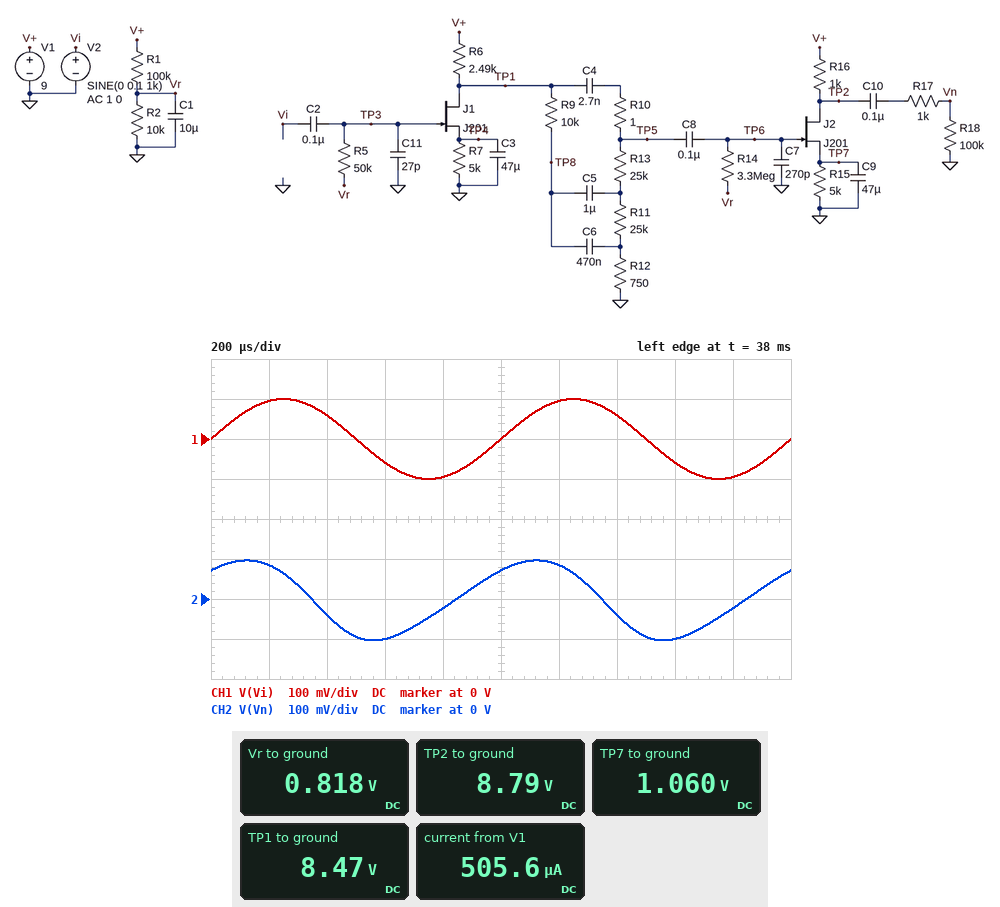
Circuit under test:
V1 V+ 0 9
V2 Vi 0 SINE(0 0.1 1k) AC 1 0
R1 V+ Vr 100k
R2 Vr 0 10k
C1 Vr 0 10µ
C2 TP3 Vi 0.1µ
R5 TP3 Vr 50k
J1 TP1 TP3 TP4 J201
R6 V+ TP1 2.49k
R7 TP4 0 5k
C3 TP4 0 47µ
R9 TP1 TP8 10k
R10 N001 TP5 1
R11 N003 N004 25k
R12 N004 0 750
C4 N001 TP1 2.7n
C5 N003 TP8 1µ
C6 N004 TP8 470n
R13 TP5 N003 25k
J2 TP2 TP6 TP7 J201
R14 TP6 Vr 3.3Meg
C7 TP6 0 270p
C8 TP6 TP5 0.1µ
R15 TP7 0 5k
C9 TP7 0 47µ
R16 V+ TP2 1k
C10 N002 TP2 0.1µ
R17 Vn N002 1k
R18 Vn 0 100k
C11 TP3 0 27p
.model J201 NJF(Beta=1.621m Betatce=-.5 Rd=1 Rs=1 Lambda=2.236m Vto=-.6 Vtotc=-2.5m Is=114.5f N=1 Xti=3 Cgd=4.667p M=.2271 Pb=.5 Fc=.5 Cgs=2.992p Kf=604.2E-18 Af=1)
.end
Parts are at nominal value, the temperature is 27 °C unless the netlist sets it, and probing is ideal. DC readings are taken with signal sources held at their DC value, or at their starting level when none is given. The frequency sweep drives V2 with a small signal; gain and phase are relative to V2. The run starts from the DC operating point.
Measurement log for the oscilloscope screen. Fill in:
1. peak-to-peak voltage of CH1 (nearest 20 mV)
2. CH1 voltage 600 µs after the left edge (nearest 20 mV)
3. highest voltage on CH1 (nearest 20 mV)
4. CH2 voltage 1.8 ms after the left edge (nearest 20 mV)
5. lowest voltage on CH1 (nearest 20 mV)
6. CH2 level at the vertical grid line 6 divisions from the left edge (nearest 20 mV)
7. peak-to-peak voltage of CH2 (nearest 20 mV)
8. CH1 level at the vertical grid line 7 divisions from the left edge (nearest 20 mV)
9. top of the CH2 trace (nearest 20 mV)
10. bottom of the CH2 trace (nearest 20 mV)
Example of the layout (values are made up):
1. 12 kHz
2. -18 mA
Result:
1. 200 mV
2. -60 mV
3. 100 mV
4. -20 mV
5. -100 mV
6. 80 mV
7. 200 mV
8. 60 mV
9. 100 mV
10. -100 mV
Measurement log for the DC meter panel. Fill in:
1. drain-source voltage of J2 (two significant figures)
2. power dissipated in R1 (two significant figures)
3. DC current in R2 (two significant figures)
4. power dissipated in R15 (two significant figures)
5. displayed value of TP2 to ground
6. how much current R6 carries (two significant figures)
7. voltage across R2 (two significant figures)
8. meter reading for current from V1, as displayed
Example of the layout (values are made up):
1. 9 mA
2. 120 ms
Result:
1. 7.7 V
2. 670 µW
3. 82 µA
4. 220 µW
5. 8.79 V
6. 210 µA
7. 820 mV
8. 505.6 µA
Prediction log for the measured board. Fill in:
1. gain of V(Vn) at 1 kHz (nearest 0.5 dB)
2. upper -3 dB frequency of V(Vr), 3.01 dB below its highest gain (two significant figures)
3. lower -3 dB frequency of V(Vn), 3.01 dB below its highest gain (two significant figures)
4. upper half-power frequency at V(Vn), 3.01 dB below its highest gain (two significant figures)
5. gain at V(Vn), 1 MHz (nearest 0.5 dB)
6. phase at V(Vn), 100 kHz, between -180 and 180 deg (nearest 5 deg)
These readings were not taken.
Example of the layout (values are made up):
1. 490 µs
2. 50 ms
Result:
1. 0 dB
2. 35 Hz
3. 2.0 kHz
4. 340 kHz
5. -2.5 dB
6. -15 deg
